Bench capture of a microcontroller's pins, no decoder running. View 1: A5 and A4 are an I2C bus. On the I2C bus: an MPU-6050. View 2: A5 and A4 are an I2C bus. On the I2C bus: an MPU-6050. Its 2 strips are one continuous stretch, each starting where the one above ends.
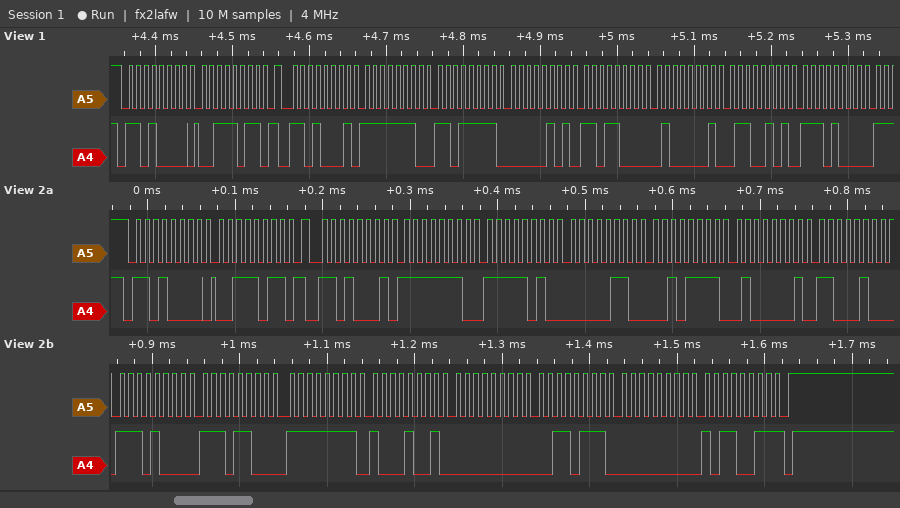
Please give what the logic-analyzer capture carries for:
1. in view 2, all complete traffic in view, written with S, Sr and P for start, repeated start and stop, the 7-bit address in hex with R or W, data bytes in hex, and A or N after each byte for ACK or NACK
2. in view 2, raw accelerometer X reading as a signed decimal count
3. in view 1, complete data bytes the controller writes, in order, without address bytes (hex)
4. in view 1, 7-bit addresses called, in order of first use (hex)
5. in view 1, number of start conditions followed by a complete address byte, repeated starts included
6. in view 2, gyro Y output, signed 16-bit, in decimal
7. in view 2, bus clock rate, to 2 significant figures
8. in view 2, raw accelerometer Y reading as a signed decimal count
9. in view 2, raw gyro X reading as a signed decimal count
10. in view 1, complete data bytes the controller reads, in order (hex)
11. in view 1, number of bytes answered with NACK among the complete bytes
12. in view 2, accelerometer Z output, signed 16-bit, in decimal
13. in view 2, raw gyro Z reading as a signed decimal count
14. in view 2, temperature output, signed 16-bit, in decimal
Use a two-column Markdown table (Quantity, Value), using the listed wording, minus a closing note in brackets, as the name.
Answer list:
| Quantity | Value |
|---|---|
| in view 2, all complete traffic in view, written with S, Sr and P for start, repeated start and stop, the 7-bit address in hex with R or W, data bytes in hex, and A or N after each byte for ACK or NACK | S 68W A 3B A Sr 68R A FE A FA A 06 A 2F A 41 A C4 A E8 A EC A FF A 89 A 00 A 37 A 00 A B3 N P |
| in view 2, raw accelerometer X reading as a signed decimal count | -262 |
| in view 1, complete data bytes the controller writes, in order, without address bytes | 3B |
| in view 1, 7-bit addresses called, in order of first use | 0x68 |
| in view 1, number of start conditions followed by a complete address byte, repeated starts included | 2 |
| in view 2, gyro Y output, signed 16-bit, in decimal | 55 |
| in view 2, bus clock rate, to 2 significant figures | 100 kHz |
| in view 2, raw accelerometer Y reading as a signed decimal count | 1583 |
| in view 2, raw gyro X reading as a signed decimal count | -119 |
| in view 1, complete data bytes the controller reads, in order | FE DF 05 D8 41 65 E8 |
| in view 1, number of bytes answered with NACK among the complete bytes | 0 |
| in view 2, accelerometer Z output, signed 16-bit, in decimal | 16836 |
| in view 2, raw gyro Z reading as a signed decimal count | 179 |
| in view 2, temperature output, signed 16-bit, in decimal | -5908 |
